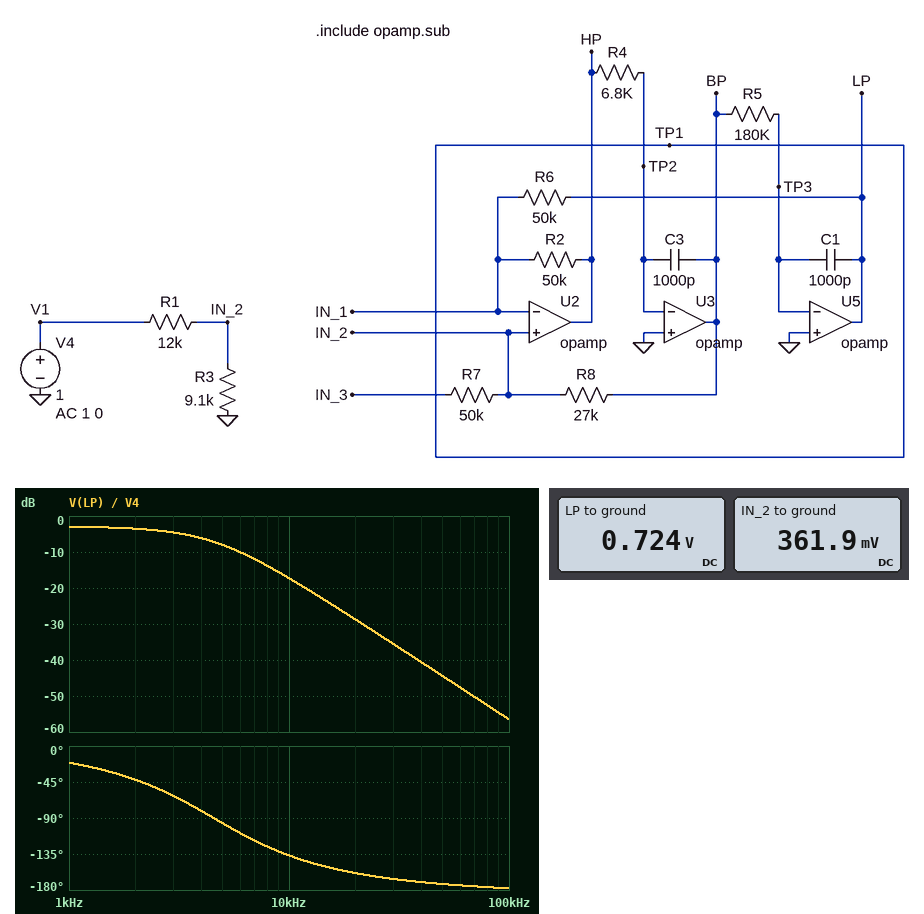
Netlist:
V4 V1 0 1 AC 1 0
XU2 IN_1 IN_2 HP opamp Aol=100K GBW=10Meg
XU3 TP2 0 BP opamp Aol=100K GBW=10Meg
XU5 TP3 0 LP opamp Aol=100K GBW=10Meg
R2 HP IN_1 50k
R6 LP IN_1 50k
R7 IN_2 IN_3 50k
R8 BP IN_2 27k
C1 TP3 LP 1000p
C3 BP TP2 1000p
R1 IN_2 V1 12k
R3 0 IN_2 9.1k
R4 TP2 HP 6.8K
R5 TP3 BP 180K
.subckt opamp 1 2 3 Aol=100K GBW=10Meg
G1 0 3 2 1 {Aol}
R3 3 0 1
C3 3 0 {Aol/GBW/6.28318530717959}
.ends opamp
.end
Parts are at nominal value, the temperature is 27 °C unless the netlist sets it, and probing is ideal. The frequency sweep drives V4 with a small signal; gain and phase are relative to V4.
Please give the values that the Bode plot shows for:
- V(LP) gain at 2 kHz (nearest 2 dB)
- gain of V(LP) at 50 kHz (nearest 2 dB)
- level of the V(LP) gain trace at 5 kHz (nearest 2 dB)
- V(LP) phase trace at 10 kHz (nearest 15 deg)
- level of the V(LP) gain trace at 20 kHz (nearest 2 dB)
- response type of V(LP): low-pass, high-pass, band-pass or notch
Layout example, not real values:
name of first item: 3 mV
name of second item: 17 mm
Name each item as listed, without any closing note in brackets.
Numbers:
V(LP) gain at 2 kHz: -4 dB
gain of V(LP) at 50 kHz: -44 dB
level of the V(LP) gain trace at 5 kHz: -8 dB
V(LP) phase trace at 10 kHz: -135 deg
level of the V(LP) gain trace at 20 kHz: -28 dB
response type of V(LP): low-pass, high-pass, band-pass or notch: low-pass
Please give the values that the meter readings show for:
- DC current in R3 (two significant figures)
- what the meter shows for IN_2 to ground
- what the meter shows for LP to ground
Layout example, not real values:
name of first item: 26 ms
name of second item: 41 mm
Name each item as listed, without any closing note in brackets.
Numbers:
DC current in R3: 40 µA
what the meter shows for IN_2 to ground: 361.9 mV
what the meter shows for LP to ground: 0.724 V
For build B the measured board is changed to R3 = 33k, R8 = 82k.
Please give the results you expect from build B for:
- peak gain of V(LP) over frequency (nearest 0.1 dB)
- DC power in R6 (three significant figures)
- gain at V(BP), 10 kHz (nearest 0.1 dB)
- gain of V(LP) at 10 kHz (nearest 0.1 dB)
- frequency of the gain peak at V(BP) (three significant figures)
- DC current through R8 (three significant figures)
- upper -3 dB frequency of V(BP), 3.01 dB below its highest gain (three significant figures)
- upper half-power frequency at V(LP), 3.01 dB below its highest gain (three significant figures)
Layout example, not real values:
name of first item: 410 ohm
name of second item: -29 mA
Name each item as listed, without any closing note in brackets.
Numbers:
peak gain of V(LP) over frequency: 3.7 dB
DC power in R6: 8.77 µW
gain at V(BP), 10 kHz: 10.6 dB
gain of V(LP) at 10 kHz: -10.5 dB
frequency of the gain peak at V(BP): 4.55 kHz
DC current through R8: 8.08 µA
upper -3 dB frequency of V(BP), 3.01 dB below its highest gain: 7.34 kHz
upper half-power frequency at V(LP), 3.01 dB below its highest gain: 5.32 kHz
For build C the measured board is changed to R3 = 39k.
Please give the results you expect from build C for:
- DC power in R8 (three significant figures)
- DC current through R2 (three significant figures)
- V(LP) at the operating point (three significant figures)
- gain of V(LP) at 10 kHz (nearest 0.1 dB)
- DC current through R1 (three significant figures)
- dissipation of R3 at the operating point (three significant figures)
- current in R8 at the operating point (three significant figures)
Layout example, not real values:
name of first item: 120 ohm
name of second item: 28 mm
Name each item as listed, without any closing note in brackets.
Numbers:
DC power in R8: 12.1 µW
DC current through R2: 11.4 µA
V(LP) at the operating point: 1.14 V
gain of V(LP) at 10 kHz: -15.6 dB
DC current through R1: 35.8 µA
dissipation of R3 at the operating point: 8.35 µW
current in R8 at the operating point: 21.1 µA
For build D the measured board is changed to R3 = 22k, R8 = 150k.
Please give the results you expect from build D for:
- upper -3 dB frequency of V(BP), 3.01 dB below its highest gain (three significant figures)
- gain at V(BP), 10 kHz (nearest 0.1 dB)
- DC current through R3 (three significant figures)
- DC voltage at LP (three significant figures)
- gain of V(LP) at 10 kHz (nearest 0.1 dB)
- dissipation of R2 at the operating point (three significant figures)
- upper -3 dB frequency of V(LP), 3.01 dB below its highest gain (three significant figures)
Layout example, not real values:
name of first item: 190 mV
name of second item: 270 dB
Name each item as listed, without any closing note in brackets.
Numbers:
upper -3 dB frequency of V(BP), 3.01 dB below its highest gain: 5.83 kHz
gain at V(BP), 10 kHz: 10.8 dB
DC current through R3: 28.0 µA
DC voltage at LP: 1.23 V
gain of V(LP) at 10 kHz: -10.2 dB
dissipation of R2 at the operating point: 7.57 µW
upper -3 dB frequency of V(LP), 3.01 dB below its highest gain: 5.30 kHz
